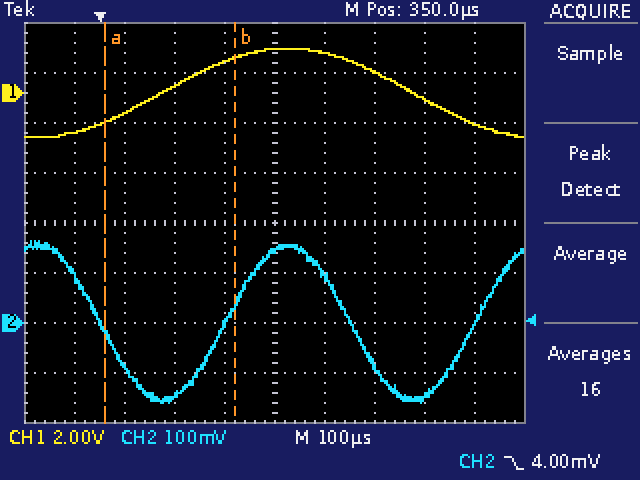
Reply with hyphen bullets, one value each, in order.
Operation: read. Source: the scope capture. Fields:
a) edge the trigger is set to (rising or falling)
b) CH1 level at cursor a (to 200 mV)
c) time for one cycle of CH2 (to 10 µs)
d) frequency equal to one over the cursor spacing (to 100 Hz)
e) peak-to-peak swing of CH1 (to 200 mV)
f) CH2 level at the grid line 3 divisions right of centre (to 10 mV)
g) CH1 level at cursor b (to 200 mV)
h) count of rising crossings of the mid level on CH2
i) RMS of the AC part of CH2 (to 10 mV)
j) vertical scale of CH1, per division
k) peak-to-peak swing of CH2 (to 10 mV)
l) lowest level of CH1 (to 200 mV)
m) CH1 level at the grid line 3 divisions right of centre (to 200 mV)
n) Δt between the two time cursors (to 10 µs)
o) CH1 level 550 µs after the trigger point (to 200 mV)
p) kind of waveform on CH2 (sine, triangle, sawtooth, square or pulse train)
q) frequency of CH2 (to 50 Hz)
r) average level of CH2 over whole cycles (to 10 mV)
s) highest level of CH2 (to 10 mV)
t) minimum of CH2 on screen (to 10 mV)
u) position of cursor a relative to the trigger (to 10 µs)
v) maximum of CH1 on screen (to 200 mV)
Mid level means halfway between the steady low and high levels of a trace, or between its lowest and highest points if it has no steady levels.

- falling
- -1.2 V
- 500 µs
- 3.8 kHz
- 3.6 V
- -150 mV
- 1.4 V
- 2
- 110 mV
- 2 V
- 320 mV
- -1.8 V
- -200 mV
- 260 µs
- 800 mV
- sine
- 2.00 kHz
- 0 mV
- 160 mV
- -160 mV
- +10 µs
- 1.8 V
